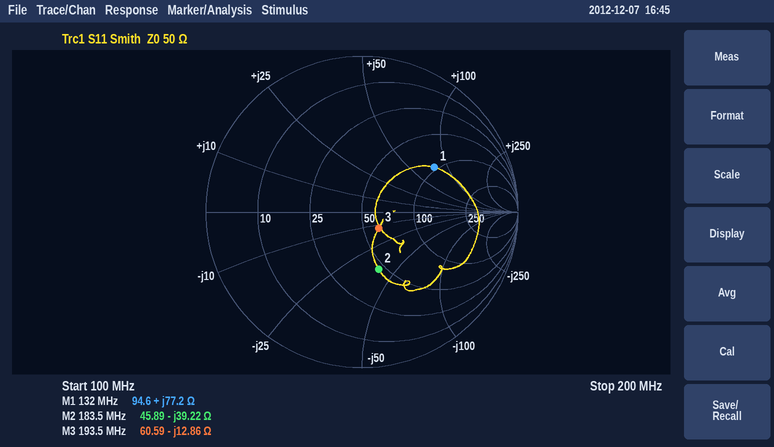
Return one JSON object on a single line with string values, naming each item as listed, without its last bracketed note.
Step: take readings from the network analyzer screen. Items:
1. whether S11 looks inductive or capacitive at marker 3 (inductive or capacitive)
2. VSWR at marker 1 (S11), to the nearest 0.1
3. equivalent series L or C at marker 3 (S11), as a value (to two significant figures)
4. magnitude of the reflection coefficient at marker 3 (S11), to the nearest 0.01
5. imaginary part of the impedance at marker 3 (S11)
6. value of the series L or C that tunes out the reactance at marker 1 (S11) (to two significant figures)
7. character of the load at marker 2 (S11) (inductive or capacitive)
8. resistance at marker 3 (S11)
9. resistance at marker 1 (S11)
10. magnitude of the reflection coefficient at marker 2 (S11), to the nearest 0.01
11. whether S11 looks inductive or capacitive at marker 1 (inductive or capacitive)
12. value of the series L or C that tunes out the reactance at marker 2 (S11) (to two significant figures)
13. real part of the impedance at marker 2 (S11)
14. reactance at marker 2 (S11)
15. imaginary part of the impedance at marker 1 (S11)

{"whether S11 looks inductive or capacitive at marker 3": "capacitive", "VSWR at marker 1 (S11), to the nearest 0.1": "3.4", "equivalent series L or C at marker 3 (S11), as a value": "64 pF", "magnitude of the reflection coefficient at marker 3 (S11), to the nearest 0.01": "0.15", "imaginary part of the impedance at marker 3": "-12.86 Ω", "value of the series L or C that tunes out the reactance at marker 1 (S11)": "16 pF", "character of the load at marker 2 (S11)": "capacitive", "resistance at marker 3": "60.59 Ω", "resistance at marker 1": "94.6 Ω", "magnitude of the reflection coefficient at marker 2 (S11), to the nearest 0.01": "0.38", "whether S11 looks inductive or capacitive at marker 1": "inductive", "value of the series L or C that tunes out the reactance at marker 2 (S11)": "34 nH", "real part of the impedance at marker 2": "45.89 Ω", "reactance at marker 2": "-39.22 Ω", "imaginary part of the impedance at marker 1": "+77.2 Ω"}
